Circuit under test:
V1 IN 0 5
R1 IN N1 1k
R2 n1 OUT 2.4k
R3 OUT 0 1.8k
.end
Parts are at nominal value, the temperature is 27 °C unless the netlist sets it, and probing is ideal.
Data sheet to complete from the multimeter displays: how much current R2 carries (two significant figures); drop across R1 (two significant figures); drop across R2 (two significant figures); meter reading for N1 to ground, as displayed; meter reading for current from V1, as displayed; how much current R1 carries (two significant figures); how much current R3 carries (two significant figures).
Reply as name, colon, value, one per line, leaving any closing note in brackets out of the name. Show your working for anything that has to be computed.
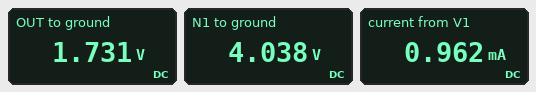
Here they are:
how much current R2 carries: (4.038 V - 1.731 V) / 2.4 kΩ = 960 µA
drop across R1: 5 V - 4.038 V = 960 mV
drop across R2: 4.038 V - 1.731 V = 2.3 V
meter reading for N1 to ground, as displayed: 4.038 V
meter reading for current from V1, as displayed: 0.962 mA
how much current R1 carries: (5 V - 4.038 V) / 1 kΩ = 960 µA
how much current R3 carries: (1.731 V) / 1.8 kΩ = 960 µA
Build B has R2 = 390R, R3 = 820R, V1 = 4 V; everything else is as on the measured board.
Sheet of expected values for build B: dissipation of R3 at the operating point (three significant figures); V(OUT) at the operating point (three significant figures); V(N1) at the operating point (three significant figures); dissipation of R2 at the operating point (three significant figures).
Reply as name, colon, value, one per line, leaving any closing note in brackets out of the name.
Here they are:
dissipation of R3 at the operating point: 2.69 mW
V(OUT) at the operating point: 1.48 V
V(N1) at the operating point: 2.19 V
dissipation of R2 at the operating point: 1.28 mW
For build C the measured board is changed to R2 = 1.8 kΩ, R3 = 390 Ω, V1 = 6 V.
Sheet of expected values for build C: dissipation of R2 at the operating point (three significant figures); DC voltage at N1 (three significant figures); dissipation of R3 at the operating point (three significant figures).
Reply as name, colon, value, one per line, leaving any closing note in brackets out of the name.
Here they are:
dissipation of R2 at the operating point: 6.37 mW
DC voltage at N1: 4.12 V
dissipation of R3 at the operating point: 1.38 mW
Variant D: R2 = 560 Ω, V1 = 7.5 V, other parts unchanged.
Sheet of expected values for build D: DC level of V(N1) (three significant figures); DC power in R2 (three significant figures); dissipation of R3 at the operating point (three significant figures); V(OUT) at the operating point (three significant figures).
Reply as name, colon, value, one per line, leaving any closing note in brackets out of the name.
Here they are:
DC level of V(N1): 5.27 V
DC power in R2: 2.79 mW
dissipation of R3 at the operating point: 8.97 mW
V(OUT) at the operating point: 4.02 V
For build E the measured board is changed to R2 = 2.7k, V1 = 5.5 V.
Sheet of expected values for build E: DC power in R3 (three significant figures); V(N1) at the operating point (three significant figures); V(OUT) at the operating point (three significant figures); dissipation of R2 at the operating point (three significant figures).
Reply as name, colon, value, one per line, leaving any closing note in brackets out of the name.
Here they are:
DC power in R3: 1.80 mW
V(N1) at the operating point: 4.50 V
V(OUT) at the operating point: 1.80 V
dissipation of R2 at the operating point: 2.70 mW
